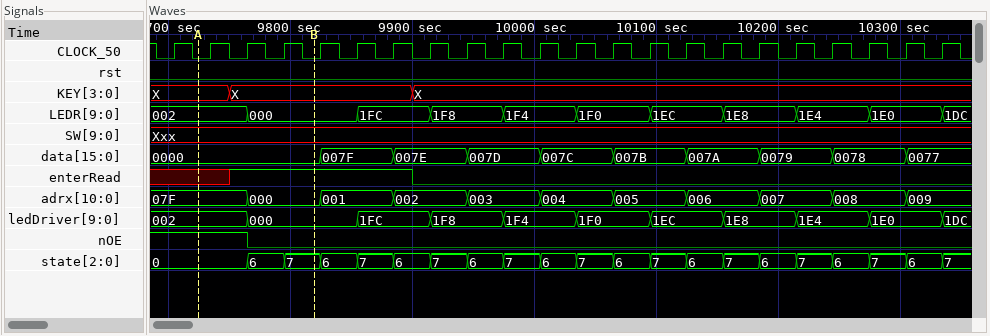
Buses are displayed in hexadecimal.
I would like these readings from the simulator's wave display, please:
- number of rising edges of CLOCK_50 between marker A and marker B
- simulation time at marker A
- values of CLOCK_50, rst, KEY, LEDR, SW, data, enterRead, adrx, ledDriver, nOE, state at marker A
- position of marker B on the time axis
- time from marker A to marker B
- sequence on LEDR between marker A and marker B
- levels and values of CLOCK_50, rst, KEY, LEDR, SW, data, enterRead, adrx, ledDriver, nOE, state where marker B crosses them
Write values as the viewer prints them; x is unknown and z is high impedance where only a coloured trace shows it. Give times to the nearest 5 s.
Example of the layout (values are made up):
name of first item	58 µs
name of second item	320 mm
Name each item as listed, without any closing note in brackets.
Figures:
number of rising edges of CLOCK_50 between marker A and marker B	3
simulation time at marker A	9725 s
values of CLOCK_50, rst, KEY, LEDR, SW, data, enterRead, adrx, ledDriver, nOE, state at marker A	CLOCK_50=0, rst=0, KEY=X, LEDR=002, SW=Xxx, data=0000, enterRead=x, adrx=07F, ledDriver=002, nOE=1, state=0
position of marker B on the time axis	9820 s
time from marker A to marker B	95 s
sequence on LEDR between marker A and marker B	002, 000
levels and values of CLOCK_50, rst, KEY, LEDR, SW, data, enterRead, adrx, ledDriver, nOE, state where marker B crosses them	CLOCK_50=0, rst=0, KEY=X, LEDR=000, SW=Xxx, data=0000, enterRead=1, adrx=000, ledDriver=000, nOE=0, state=7
